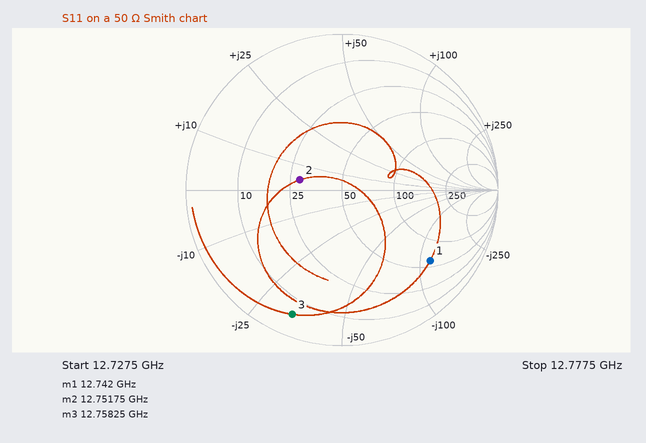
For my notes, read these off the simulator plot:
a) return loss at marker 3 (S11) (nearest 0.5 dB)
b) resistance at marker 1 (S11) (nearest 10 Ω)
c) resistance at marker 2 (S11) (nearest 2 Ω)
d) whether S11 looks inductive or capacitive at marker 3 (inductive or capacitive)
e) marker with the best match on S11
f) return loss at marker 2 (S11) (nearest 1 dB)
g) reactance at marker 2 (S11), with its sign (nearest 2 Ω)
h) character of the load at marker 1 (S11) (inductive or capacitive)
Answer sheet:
1.5 dB
60 Ω
28 Ω
capacitive
marker 2
11 dB
+4 Ω
capacitive
